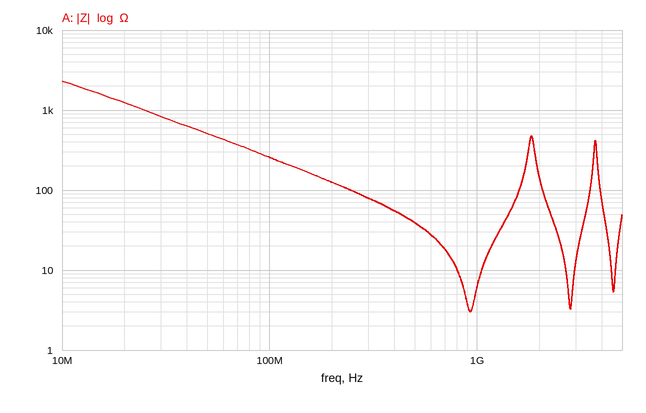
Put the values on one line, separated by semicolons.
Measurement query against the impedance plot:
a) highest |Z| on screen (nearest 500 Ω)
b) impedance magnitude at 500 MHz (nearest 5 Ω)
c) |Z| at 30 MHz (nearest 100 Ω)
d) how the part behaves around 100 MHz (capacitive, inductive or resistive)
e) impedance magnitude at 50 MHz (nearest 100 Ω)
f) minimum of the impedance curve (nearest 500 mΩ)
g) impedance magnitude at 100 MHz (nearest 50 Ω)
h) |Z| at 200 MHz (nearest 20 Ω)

2.5 kΩ; 40 Ω; 800 Ω; capacitive; 500 Ω; 3.0 Ω; 250 Ω; 120 Ω
